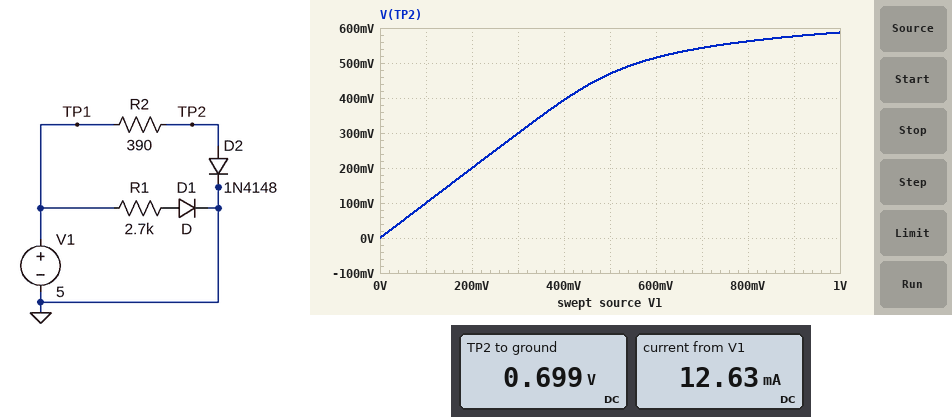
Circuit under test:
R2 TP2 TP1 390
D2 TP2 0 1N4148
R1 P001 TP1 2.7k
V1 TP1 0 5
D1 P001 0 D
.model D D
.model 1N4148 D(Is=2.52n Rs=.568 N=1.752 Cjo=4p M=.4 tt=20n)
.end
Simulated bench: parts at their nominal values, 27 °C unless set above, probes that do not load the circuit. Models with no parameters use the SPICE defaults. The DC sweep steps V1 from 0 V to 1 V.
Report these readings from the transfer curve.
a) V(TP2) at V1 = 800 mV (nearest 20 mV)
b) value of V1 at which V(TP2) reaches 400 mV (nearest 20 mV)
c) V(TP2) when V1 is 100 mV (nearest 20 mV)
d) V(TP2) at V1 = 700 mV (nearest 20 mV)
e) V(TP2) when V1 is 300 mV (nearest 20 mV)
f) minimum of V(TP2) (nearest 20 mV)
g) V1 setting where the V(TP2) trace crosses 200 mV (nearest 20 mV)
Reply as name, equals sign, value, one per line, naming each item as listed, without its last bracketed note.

V(TP2) at V1 = 800 mV = 560 mV
value of V1 at which V(TP2) reaches 400 mV = 400 mV
V(TP2) when V1 is 100 mV = 100 mV
V(TP2) at V1 = 700 mV = 540 mV
V(TP2) when V1 is 300 mV = 300 mV
minimum of V(TP2) = 0 V
V1 setting where the V(TP2) trace crosses 200 mV = 200 mV
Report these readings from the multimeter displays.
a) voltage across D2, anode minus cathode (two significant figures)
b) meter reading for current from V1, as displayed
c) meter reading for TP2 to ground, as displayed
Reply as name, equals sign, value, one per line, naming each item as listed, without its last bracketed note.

voltage across D2, anode minus cathode = 700 mV
meter reading for current from V1, as displayed = 12.63 mA
meter reading for TP2 to ground, as displayed = 0.699 V
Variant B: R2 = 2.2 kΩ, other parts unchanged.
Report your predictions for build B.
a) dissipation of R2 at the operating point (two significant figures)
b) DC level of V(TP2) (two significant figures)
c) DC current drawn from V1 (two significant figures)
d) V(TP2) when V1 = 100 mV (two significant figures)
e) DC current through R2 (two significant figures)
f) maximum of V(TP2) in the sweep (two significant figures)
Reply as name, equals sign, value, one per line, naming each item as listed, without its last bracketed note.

dissipation of R2 at the operating point = 8.7 mW
DC level of V(TP2) = 620 mV
DC current drawn from V1 = 3.6 mA
V(TP2) when V1 = 100 mV = 100 mV
DC current through R2 = 2.0 mA
maximum of V(TP2) in the sweep = 520 mV
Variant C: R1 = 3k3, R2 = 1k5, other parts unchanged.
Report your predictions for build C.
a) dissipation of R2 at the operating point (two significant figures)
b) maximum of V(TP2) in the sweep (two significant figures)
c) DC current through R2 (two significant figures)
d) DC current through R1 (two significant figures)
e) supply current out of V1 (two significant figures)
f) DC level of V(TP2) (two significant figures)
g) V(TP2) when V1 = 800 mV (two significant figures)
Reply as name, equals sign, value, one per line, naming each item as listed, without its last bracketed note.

dissipation of R2 at the operating point = 13 mW
maximum of V(TP2) in the sweep = 530 mV
DC current through R2 = 2.9 mA
DC current through R1 = 1.3 mA
supply current out of V1 = 4.2 mA
DC level of V(TP2) = 630 mV
V(TP2) when V1 = 800 mV = 510 mV
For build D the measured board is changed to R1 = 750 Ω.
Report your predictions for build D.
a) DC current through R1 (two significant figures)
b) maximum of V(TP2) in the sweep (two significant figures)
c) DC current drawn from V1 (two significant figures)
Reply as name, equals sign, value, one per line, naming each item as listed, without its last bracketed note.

DC current through R1 = 5.7 mA
maximum of V(TP2) in the sweep = 590 mV
DC current drawn from V1 = 17 mA
